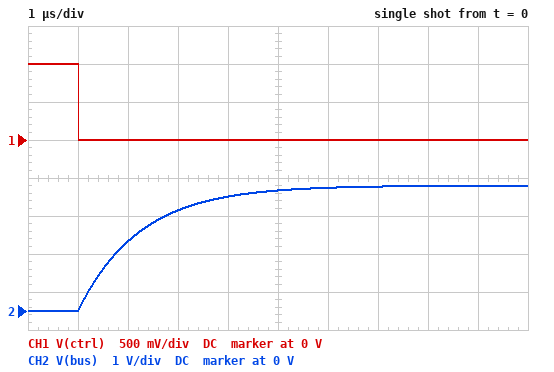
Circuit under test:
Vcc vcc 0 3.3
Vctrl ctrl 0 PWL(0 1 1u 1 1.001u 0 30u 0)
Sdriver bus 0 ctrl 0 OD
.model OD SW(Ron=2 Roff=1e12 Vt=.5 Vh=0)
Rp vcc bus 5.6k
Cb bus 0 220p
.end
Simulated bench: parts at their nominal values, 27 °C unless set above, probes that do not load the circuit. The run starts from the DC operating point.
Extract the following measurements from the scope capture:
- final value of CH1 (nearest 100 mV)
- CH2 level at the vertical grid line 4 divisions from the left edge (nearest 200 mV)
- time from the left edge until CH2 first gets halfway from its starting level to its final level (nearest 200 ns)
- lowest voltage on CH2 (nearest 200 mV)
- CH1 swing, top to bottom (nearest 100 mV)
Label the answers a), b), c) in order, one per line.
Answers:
a) 0 V
b) 3.0 V
c) 1.8 µs
d) 0 V
e) 1.0 V
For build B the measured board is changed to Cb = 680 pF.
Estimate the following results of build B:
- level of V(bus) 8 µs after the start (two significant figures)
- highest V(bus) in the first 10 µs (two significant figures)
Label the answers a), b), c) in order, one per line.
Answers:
a) 2.8 V
b) 3.0 V
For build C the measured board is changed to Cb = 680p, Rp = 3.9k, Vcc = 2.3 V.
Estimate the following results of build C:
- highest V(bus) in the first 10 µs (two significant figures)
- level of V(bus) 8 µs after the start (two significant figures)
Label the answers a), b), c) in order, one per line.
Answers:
a) 2.2 V
b) 2.1 V
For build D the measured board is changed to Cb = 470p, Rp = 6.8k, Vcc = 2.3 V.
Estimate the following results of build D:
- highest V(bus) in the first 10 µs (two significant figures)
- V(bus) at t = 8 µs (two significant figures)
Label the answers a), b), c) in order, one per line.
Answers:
a) 2.2 V
b) 2.0 V
